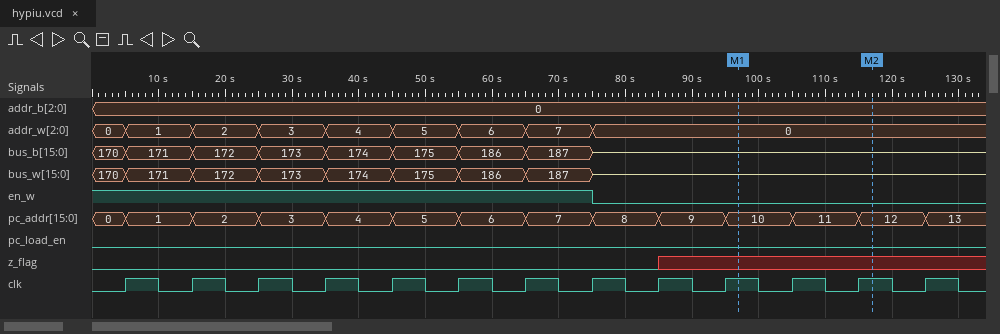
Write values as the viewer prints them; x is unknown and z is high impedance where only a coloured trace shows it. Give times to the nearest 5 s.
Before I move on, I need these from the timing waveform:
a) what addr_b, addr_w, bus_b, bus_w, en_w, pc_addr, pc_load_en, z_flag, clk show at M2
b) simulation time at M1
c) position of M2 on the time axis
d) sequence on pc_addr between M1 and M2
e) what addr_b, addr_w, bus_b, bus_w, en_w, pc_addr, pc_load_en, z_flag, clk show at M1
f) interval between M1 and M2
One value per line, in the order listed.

addr_b=0, addr_w=0, bus_b=z, bus_w=z, en_w=0, pc_addr=12, pc_load_en=0, z_flag=x, clk=1
95 s
115 s
10, 11, 12
addr_b=0, addr_w=0, bus_b=z, bus_w=z, en_w=0, pc_addr=10, pc_load_en=0, z_flag=x, clk=1
20 s
